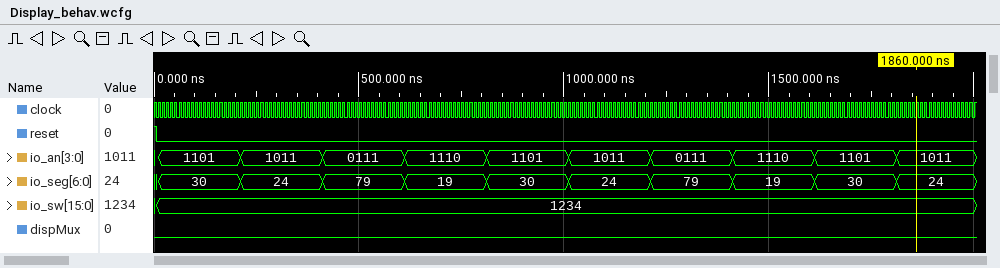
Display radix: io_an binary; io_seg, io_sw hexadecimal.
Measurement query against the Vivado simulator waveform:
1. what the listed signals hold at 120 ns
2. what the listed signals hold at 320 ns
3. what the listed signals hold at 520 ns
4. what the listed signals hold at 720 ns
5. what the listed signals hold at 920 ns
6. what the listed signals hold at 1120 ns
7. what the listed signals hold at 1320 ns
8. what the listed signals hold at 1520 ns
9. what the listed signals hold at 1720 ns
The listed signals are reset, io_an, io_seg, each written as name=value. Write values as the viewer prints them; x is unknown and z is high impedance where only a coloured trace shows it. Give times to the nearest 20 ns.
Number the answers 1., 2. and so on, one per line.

1. reset=0, io_an=1101, io_seg=30
2. reset=0, io_an=1011, io_seg=24
3. reset=0, io_an=0111, io_seg=79
4. reset=0, io_an=1110, io_seg=19
5. reset=0, io_an=1101, io_seg=30
6. reset=0, io_an=1011, io_seg=24
7. reset=0, io_an=0111, io_seg=79
8. reset=0, io_an=1110, io_seg=19
9. reset=0, io_an=1101, io_seg=30
